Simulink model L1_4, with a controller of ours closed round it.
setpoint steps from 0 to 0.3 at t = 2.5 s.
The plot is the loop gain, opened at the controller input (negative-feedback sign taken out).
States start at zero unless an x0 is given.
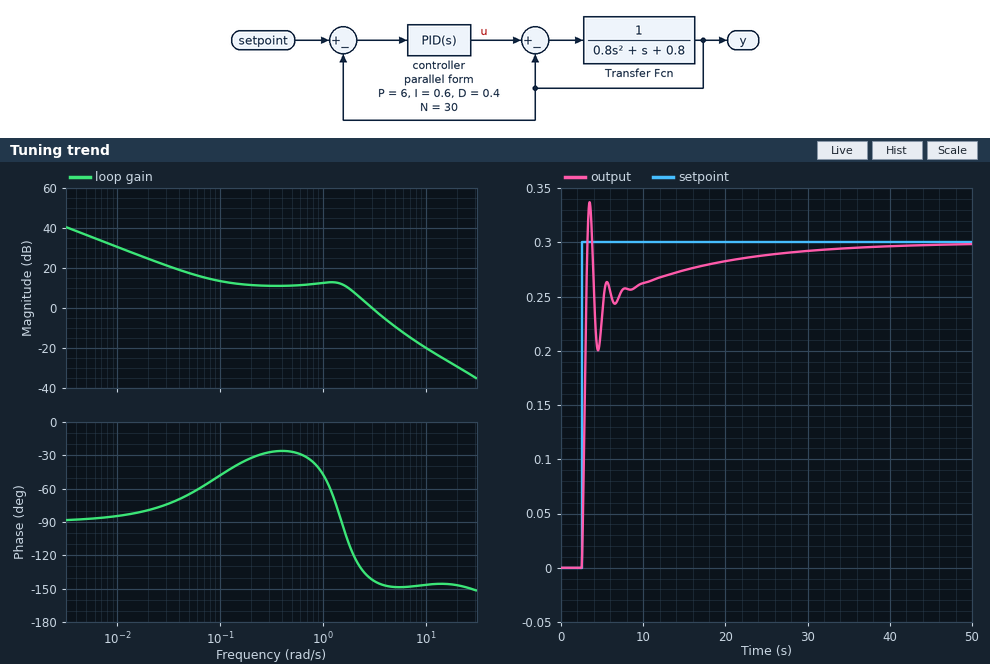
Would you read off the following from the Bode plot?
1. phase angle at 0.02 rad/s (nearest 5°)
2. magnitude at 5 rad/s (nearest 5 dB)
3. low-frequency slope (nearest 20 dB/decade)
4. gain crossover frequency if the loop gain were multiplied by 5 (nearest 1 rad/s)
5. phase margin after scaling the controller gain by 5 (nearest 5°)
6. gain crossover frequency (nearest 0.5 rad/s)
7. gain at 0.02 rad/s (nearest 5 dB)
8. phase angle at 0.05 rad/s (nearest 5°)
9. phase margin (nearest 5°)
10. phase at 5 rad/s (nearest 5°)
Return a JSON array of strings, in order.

["-80°", "-10 dB", "-20 dB/decade", "7 rad/s", "30°", "3.0 rad/s", "25 dB", "-65°", "40°", "-150°"]
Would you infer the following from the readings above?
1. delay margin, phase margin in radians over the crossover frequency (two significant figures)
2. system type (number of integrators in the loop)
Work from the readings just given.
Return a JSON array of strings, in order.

["0.23 s", "1"]
